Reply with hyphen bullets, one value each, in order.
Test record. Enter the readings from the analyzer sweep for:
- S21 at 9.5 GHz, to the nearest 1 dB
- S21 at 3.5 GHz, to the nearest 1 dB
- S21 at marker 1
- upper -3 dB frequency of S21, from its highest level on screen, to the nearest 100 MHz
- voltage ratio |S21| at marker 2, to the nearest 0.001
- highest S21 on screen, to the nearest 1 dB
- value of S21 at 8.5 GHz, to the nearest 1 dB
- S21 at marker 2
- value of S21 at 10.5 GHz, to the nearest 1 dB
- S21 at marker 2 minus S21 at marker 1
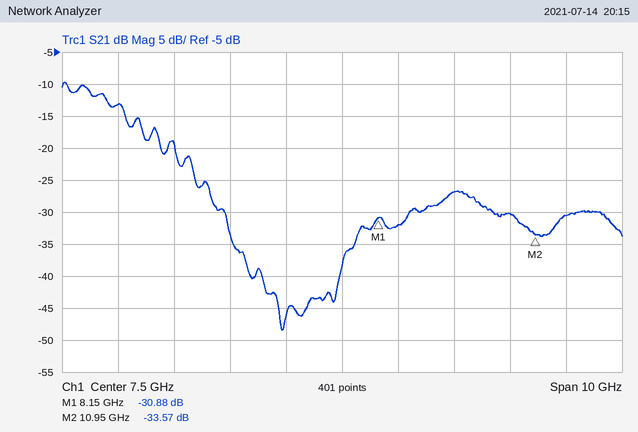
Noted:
- -27 dB
- -13 dB
- -30.88 dB
- 3.3 GHz
- 0.021
- -10 dB
- -32 dB
- -33.57 dB
- -30 dB
- -2.69 dB
